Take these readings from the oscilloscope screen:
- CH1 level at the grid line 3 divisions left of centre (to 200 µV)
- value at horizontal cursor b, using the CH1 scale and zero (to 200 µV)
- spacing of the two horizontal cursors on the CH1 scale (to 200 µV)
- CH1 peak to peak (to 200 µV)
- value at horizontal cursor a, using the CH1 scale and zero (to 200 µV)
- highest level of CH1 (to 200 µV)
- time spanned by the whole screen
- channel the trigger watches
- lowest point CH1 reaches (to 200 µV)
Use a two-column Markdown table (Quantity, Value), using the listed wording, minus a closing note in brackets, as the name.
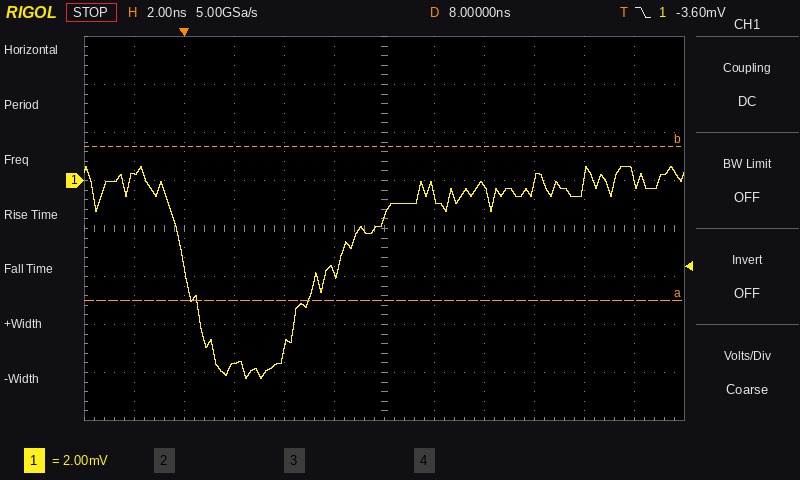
| Quantity | Value |
|---|---|
| CH1 level at the grid line 3 divisions left of centre | -7.6 mV |
| value at horizontal cursor b, using the CH1 scale and zero | 1.4 mV |
| spacing of the two horizontal cursors on the CH1 scale | 6.4 mV |
| CH1 peak to peak | 8.8 mV |
| value at horizontal cursor a, using the CH1 scale and zero | -5.0 mV |
| highest level of CH1 | 600 µV |
| time spanned by the whole screen | 24 ns |
| channel the trigger watches | CH1 |
| lowest point CH1 reaches | -8.2 mV |
